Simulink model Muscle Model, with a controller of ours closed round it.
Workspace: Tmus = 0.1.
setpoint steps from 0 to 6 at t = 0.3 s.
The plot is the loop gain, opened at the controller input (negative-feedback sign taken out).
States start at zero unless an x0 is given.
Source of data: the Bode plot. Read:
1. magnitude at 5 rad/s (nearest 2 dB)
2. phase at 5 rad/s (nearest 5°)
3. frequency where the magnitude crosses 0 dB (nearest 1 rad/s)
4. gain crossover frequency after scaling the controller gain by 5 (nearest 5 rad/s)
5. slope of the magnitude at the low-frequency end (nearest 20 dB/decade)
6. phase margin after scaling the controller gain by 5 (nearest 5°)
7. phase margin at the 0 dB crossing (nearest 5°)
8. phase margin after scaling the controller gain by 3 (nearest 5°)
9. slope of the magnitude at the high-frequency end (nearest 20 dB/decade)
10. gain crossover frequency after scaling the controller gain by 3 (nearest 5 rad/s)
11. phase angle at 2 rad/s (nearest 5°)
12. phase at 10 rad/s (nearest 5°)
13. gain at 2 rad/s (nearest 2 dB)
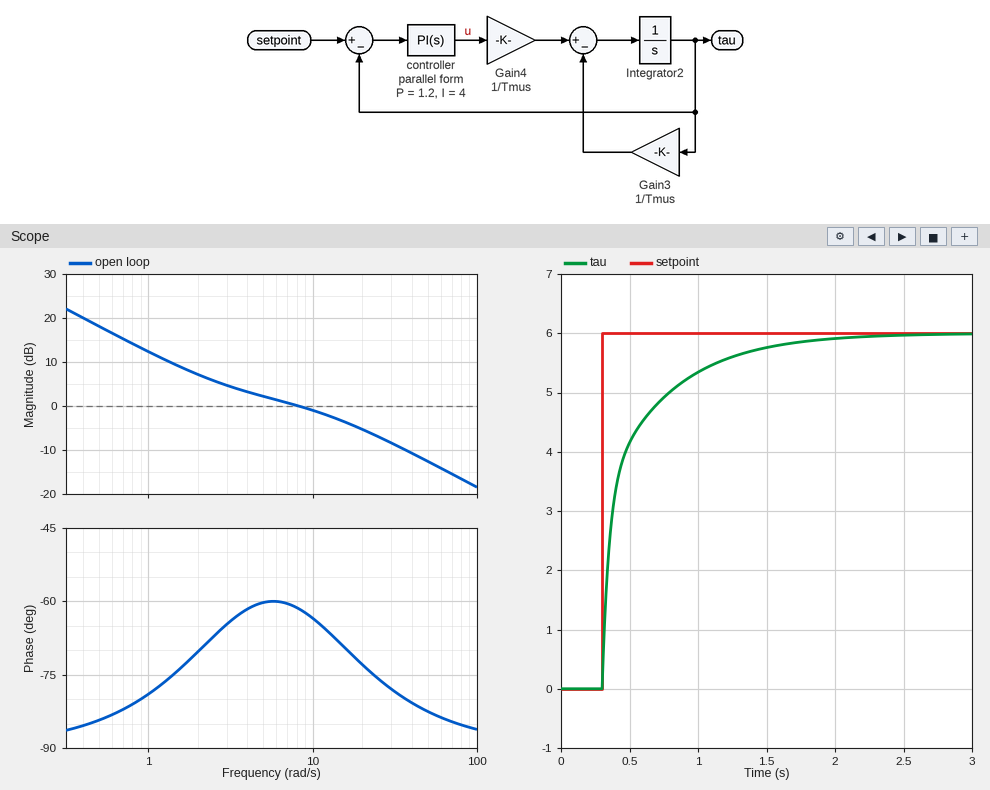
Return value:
2 dB
-60°
8 rad/s
60 rad/s
-20 dB/decade
95°
120°
100°
-20 dB/decade
35 rad/s
-70°
-65°
8 dB
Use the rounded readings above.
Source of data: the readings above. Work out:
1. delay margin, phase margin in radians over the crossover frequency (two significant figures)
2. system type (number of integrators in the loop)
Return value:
0.26 s
1
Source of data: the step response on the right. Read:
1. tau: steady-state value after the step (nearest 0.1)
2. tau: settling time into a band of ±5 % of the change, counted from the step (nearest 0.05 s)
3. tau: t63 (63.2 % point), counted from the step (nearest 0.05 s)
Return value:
6.0
1.10 s
0.15 s
